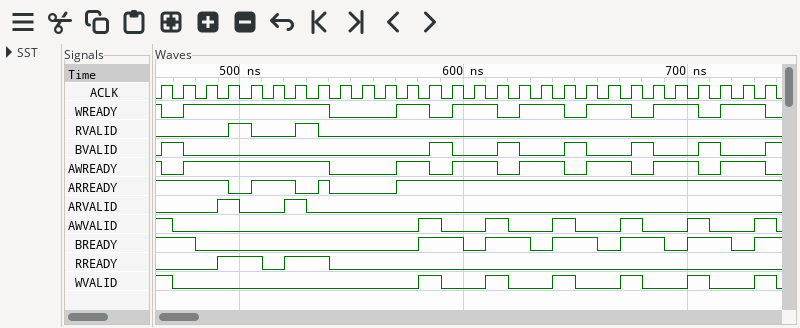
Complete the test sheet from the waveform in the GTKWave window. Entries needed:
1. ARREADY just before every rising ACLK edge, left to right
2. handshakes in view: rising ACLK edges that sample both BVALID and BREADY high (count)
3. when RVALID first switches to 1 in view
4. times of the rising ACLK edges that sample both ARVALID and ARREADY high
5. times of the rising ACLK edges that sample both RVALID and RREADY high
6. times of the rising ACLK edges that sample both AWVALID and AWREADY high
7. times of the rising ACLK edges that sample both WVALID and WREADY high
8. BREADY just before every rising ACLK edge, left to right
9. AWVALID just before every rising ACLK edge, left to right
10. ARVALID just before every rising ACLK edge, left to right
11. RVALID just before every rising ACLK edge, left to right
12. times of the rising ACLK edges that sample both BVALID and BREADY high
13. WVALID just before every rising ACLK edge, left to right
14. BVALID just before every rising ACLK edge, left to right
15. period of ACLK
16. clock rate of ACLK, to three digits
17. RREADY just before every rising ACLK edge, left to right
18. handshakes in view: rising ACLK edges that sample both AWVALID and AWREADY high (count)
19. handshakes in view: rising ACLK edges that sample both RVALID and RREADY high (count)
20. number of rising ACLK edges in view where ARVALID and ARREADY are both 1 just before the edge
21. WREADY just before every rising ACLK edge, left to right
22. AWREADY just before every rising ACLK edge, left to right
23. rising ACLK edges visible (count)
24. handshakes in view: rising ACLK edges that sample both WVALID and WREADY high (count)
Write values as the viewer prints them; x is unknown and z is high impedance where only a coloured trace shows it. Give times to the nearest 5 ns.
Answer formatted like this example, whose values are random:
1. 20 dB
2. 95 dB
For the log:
1. 1 1 1 1 0 1 1 0 0 0 0 1 1 1 1 1 1 1 1 1 1 1 1 1 1 1 1 1
2. 6
3. 495 ns
4. 495 ns, 525 ns
5. 505 ns, 535 ns
6. 465 ns, 585 ns, 615 ns, 645 ns, 675 ns, 705 ns, 735 ns
7. 465 ns, 585 ns, 615 ns, 645 ns, 675 ns, 705 ns, 735 ns
8. 1 1 0 0 0 0 0 0 0 0 0 0 1 1 0 1 1 0 1 1 0 1 1 0 1 1 0 1
9. 1 0 0 0 0 0 0 0 0 0 0 0 1 0 0 1 0 0 1 0 0 1 0 0 1 0 0 1
10. 0 0 0 1 0 0 1 0 0 0 0 0 0 0 0 0 0 0 0 0 0 0 0 0 0 0 0 0
11. 0 0 0 0 1 0 0 1 0 0 0 0 0 0 0 0 0 0 0 0 0 0 0 0 0 0 0 0
12. 475 ns, 595 ns, 625 ns, 655 ns, 685 ns, 715 ns
13. 1 0 0 0 0 0 0 0 0 0 0 0 1 0 0 1 0 0 1 0 0 1 0 0 1 0 0 1
14. 0 1 0 0 0 0 0 0 0 0 0 0 0 1 0 0 1 0 0 1 0 0 1 0 0 1 0 0
15. 10 ns
16. 100 MHz
17. 0 0 0 1 1 0 1 1 0 0 0 0 0 0 0 0 0 0 0 0 0 0 0 0 0 0 0 0
18. 7
19. 2
20. 2
21. 1 0 1 1 1 1 1 1 0 0 0 1 1 0 1 1 0 1 1 0 1 1 0 1 1 0 1 1
22. 1 0 1 1 1 1 1 1 0 0 0 1 1 0 1 1 0 1 1 0 1 1 0 1 1 0 1 1
23. 28
24. 7
